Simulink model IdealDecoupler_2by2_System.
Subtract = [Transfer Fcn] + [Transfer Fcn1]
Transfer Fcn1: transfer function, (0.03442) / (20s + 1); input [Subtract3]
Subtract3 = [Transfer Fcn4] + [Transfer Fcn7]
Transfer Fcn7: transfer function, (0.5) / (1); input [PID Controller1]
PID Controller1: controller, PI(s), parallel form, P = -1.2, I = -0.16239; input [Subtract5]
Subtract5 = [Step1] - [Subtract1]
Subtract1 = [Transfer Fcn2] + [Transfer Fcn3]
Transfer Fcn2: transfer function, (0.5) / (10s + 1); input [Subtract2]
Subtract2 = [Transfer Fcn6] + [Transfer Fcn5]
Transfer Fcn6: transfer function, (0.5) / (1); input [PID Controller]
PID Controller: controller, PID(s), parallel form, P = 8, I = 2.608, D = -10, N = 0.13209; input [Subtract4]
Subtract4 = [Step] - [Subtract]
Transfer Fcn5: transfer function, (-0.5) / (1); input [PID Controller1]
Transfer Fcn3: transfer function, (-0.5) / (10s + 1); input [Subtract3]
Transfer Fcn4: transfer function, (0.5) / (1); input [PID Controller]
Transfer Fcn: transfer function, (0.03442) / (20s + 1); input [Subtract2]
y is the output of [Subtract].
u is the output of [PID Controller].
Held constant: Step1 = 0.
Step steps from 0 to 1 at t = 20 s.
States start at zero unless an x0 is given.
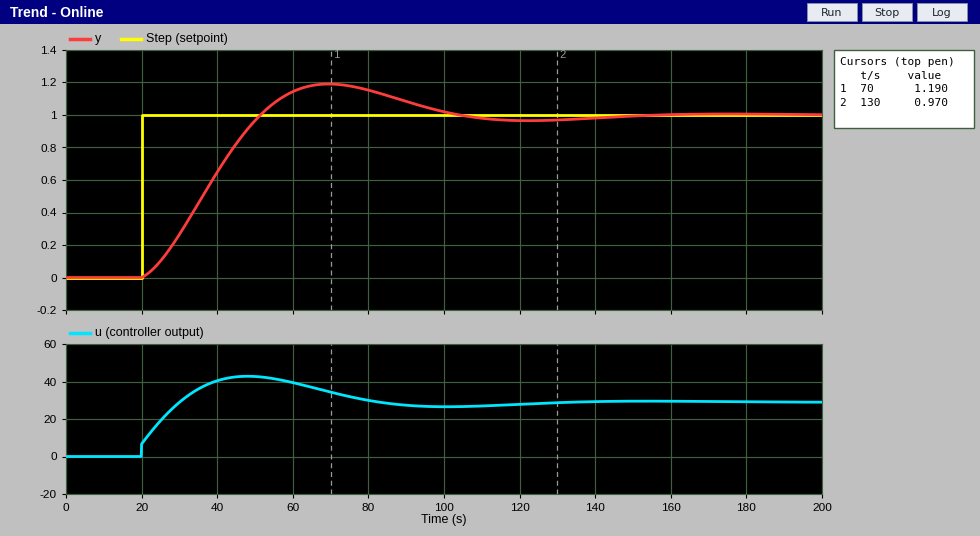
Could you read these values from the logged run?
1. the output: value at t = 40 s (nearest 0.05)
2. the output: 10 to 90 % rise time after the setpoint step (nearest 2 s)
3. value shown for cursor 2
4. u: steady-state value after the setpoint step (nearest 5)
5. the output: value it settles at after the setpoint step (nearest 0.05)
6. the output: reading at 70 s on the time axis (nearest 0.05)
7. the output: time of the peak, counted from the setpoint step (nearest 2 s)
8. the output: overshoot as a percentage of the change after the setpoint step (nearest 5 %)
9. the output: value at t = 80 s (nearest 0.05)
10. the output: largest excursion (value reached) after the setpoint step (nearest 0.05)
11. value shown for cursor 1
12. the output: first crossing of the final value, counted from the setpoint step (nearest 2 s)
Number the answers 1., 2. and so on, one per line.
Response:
1. 0.65
2. 22 s
3. 0.970
4. 30
5. 1.00
6. 1.20
7. 50 s
8. 20 %
9. 1.15
10. 1.20
11. 1.190
12. 32 s
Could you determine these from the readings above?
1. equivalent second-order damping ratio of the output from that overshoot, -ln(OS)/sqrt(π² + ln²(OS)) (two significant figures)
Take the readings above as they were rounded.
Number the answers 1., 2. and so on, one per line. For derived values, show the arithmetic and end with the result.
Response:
1. ln(0.2) = -1.609; 1.609 / sqrt(9.870 + 2.590) = 0.46
